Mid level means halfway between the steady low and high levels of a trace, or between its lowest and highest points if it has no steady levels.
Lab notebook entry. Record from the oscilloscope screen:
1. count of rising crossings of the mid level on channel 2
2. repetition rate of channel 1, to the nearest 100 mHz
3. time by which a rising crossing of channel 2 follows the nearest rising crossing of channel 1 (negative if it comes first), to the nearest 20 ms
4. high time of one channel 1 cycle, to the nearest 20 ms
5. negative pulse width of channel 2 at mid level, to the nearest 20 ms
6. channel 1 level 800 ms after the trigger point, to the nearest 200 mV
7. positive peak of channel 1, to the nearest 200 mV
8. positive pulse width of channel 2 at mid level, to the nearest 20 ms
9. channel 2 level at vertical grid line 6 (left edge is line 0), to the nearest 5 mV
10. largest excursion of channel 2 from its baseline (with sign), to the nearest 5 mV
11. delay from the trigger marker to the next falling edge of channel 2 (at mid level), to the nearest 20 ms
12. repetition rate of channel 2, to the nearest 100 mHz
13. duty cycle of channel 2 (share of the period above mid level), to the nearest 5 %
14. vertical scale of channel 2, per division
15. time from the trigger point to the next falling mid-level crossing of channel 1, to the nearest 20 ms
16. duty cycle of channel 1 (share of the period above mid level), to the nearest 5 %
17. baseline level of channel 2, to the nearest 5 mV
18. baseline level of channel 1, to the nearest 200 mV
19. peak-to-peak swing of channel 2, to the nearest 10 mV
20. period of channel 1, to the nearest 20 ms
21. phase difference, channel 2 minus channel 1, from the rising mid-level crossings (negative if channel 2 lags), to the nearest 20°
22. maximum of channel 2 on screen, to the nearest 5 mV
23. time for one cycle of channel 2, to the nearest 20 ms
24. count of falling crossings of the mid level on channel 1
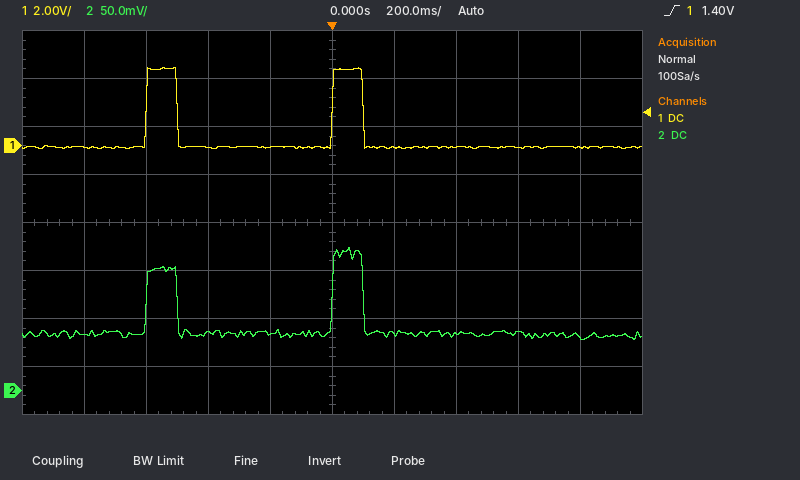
2
1.7 Hz
0 ms
100 ms
500 ms
0.0 V
3.2 V
100 ms
60 mV
+90 mV
100 ms
1.7 Hz
15 %
50 mV
100 ms
15 %
60 mV
0.0 V
100 mV
600 ms
0°
150 mV
600 ms
2
